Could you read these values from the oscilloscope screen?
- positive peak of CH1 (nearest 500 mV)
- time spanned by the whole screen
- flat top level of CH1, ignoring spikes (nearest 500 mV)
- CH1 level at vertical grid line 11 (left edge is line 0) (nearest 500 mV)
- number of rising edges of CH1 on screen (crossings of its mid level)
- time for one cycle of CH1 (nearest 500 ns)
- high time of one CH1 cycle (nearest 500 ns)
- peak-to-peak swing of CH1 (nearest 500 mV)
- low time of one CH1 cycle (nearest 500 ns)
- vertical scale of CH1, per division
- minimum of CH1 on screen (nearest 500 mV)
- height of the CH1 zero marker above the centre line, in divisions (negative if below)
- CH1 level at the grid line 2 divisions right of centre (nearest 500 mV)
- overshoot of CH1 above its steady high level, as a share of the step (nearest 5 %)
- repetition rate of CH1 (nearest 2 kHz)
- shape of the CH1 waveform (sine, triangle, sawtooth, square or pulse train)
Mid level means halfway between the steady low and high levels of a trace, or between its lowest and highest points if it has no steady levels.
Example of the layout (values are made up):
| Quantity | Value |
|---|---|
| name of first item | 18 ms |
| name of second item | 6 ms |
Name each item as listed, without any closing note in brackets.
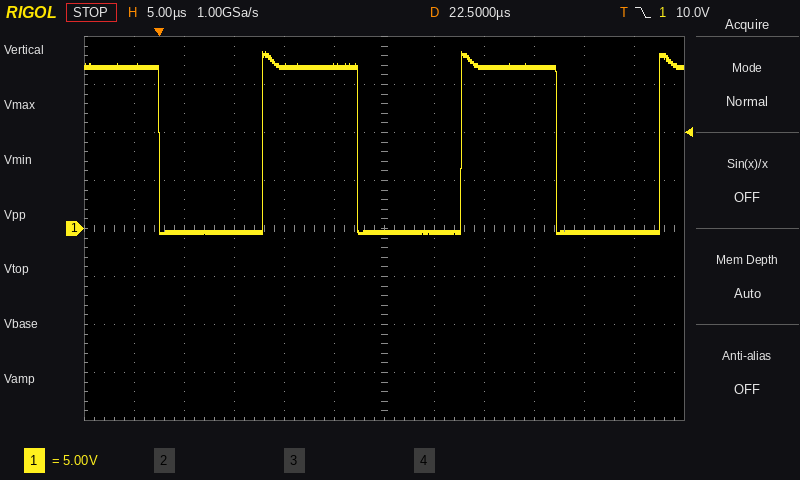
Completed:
| Quantity | Value |
|---|---|
| positive peak of CH1 | 18.5 V |
| time spanned by the whole screen | 60 µs |
| flat top level of CH1, ignoring spikes | 17.0 V |
| CH1 level at vertical grid line 11 (left edge is line 0) | -500 mV |
| number of rising edges of CH1 on screen | 3 |
| time for one cycle of CH1 | 20.0 µs |
| high time of one CH1 cycle | 9.5 µs |
| peak-to-peak swing of CH1 | 19.0 V |
| low time of one CH1 cycle | 10.5 µs |
| vertical scale of CH1, per division | 5 V |
| minimum of CH1 on screen | -500 mV |
| height of the CH1 zero marker above the centre line, in divisions | 0.0 div |
| CH1 level at the grid line 2 divisions right of centre | 17.0 V |
| overshoot of CH1 above its steady high level, as a share of the step | 10 % |
| repetition rate of CH1 | 50 kHz |
| shape of the CH1 waveform | square |
